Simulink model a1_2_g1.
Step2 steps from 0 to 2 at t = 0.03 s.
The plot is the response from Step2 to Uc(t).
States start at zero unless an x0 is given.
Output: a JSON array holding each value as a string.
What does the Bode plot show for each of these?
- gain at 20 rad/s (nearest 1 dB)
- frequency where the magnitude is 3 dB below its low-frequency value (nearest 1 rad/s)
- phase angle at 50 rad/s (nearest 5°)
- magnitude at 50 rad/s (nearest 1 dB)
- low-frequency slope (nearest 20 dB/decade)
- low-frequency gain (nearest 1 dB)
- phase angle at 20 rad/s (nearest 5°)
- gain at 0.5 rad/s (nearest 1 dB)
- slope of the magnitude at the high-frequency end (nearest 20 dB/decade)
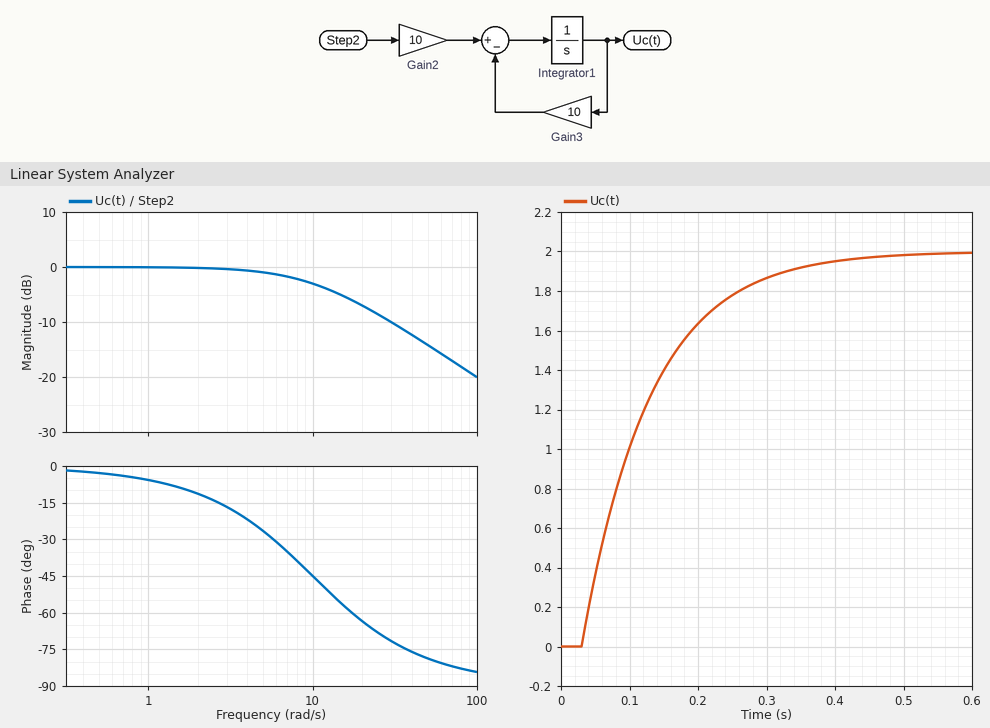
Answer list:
["-7 dB", "10 rad/s", "-80°", "-14 dB", "0 dB/decade", "0 dB", "-65°", "0 dB", "-20 dB/decade"]
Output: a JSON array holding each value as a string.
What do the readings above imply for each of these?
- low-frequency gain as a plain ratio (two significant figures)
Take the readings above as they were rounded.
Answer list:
["1.0"]
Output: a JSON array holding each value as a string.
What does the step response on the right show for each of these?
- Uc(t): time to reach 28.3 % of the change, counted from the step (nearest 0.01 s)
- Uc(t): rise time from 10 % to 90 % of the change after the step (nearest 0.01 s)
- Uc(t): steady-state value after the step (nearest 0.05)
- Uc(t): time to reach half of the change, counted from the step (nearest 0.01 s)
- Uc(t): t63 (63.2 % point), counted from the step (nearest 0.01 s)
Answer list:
["0.03 s", "0.22 s", "2.00", "0.07 s", "0.10 s"]
